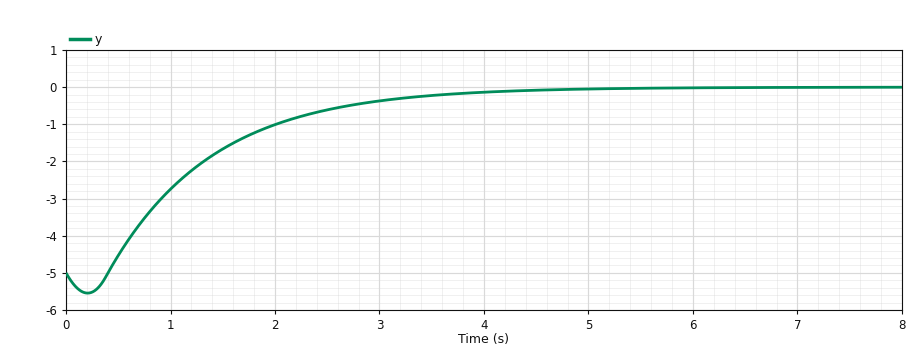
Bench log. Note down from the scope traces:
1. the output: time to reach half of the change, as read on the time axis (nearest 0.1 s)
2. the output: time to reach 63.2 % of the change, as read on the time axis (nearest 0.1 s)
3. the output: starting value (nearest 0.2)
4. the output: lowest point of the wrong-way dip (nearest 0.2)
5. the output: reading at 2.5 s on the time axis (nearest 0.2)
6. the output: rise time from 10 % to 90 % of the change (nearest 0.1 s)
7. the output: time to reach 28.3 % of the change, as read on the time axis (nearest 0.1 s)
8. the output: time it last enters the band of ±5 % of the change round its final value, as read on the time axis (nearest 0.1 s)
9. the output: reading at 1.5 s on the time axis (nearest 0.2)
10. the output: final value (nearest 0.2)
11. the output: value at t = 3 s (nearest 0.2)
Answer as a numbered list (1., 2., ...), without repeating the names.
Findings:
1. 1.1 s
2. 1.4 s
3. -5.0
4. -5.6
5. -0.6
6. 2.2 s
7. 0.7 s
8. 3.4 s
9. -1.6
10. 0.0
11. -0.4
